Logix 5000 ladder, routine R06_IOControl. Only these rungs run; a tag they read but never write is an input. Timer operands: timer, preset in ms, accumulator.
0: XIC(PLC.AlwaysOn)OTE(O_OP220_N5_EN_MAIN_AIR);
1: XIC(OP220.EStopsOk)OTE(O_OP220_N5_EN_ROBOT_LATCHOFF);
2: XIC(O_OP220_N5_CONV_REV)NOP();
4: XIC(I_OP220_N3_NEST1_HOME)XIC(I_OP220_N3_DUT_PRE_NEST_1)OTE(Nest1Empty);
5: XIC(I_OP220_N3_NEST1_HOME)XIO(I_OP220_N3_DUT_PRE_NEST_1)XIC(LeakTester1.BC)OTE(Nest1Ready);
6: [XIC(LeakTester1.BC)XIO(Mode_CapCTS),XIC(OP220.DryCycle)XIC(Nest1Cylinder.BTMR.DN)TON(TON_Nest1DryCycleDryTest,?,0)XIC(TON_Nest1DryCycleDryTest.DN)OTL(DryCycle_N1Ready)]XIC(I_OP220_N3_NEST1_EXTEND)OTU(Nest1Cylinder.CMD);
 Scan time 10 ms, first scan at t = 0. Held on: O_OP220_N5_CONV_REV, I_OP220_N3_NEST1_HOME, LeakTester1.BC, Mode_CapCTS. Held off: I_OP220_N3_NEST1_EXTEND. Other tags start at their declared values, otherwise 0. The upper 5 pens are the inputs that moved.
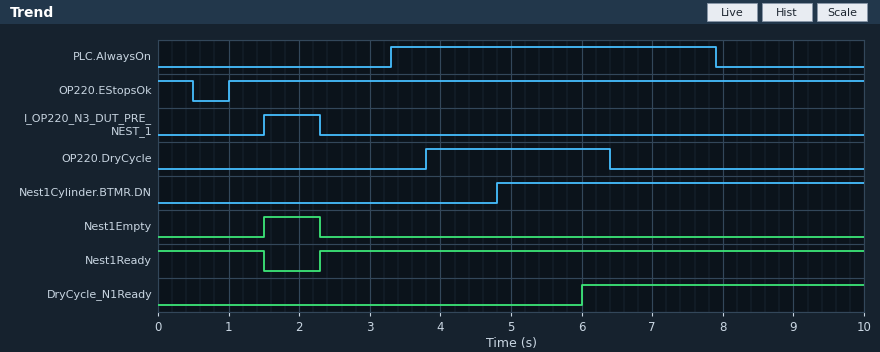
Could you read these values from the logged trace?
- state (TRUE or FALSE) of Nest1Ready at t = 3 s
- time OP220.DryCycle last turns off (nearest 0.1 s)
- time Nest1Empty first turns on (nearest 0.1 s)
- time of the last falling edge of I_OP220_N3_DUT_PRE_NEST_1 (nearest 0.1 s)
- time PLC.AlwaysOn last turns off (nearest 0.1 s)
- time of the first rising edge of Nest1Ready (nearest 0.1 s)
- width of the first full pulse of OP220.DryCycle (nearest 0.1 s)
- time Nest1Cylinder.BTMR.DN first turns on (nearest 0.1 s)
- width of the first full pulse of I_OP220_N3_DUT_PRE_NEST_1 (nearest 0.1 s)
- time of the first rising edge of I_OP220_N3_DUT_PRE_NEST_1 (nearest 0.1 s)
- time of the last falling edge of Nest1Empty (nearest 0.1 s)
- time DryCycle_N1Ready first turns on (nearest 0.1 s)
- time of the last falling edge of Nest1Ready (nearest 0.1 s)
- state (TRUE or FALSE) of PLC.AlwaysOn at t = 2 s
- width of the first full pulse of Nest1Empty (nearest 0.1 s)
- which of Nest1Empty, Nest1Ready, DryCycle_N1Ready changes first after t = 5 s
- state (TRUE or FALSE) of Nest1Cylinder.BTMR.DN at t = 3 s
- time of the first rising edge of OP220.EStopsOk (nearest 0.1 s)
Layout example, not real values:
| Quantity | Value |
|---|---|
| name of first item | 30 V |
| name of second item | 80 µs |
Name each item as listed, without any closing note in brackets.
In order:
| Quantity | Value |
|---|---|
| state (TRUE or FALSE) of Nest1Ready at t = 3 s | TRUE |
| time OP220.DryCycle last turns off | 6.4 s |
| time Nest1Empty first turns on | 1.5 s |
| time of the last falling edge of I_OP220_N3_DUT_PRE_NEST_1 | 2.3 s |
| time PLC.AlwaysOn last turns off | 7.9 s |
| time of the first rising edge of Nest1Ready | 2.3 s |
| width of the first full pulse of OP220.DryCycle | 2.6 s |
| time Nest1Cylinder.BTMR.DN first turns on | 4.8 s |
| width of the first full pulse of I_OP220_N3_DUT_PRE_NEST_1 | 0.8 s |
| time of the first rising edge of I_OP220_N3_DUT_PRE_NEST_1 | 1.5 s |
| time of the last falling edge of Nest1Empty | 2.3 s |
| time DryCycle_N1Ready first turns on | 6.0 s |
| time of the last falling edge of Nest1Ready | 1.5 s |
| state (TRUE or FALSE) of PLC.AlwaysOn at t = 2 s | FALSE |
| width of the first full pulse of Nest1Empty | 0.8 s |
| which of Nest1Empty, Nest1Ready, DryCycle_N1Ready changes first after t = 5 s | DryCycle_N1Ready |
| state (TRUE or FALSE) of Nest1Cylinder.BTMR.DN at t = 3 s | FALSE |
| time of the first rising edge of OP220.EStopsOk | 1.0 s |
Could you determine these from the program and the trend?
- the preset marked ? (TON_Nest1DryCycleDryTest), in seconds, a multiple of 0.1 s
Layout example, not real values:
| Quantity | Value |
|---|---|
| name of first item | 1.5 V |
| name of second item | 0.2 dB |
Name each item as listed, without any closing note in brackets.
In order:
| Quantity | Value |
|---|---|
| the preset marked ? (TON_Nest1DryCycleDryTest), in seconds, a multiple of 0.1 s | 1.2 s |
